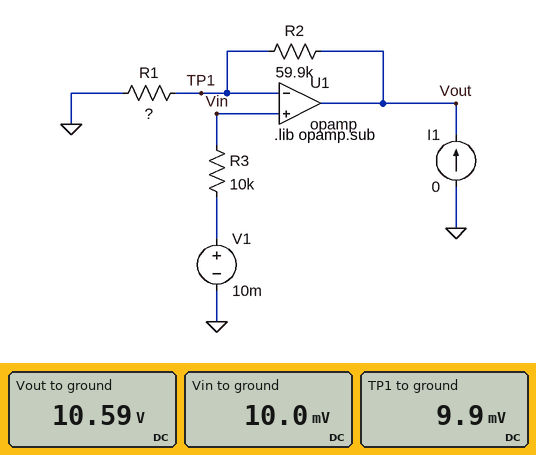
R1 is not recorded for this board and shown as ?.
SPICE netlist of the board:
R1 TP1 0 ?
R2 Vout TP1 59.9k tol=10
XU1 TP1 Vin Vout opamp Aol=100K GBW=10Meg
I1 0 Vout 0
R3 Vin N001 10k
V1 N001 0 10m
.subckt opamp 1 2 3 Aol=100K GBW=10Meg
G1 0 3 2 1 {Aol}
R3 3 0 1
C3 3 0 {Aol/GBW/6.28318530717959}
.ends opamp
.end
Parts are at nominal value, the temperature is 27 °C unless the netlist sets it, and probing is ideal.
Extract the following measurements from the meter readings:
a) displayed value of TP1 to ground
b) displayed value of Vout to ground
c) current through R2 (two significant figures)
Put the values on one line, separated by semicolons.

9.9 mV; 10.59 V; 180 µA
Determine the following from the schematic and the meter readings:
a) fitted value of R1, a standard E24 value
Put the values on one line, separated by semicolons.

56 Ω
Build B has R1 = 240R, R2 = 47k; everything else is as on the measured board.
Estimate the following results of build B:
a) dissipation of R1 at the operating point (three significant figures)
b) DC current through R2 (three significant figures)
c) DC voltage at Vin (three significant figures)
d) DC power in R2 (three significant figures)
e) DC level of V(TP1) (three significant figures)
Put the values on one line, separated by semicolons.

415 nW; 41.6 µA; 10.0 mV; 81.3 µW; 9.98 mV
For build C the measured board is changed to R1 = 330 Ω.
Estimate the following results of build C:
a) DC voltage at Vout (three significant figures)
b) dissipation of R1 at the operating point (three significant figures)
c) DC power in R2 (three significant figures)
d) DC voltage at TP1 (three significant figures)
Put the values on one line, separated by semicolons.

1.82 V; 302 nW; 54.8 µW; 9.98 mV
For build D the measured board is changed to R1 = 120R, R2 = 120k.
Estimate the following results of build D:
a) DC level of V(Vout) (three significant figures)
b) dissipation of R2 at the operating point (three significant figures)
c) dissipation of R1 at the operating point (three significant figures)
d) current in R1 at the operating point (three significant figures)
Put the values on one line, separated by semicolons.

9.91 V; 817 µW; 817 nW; 82.5 µA
